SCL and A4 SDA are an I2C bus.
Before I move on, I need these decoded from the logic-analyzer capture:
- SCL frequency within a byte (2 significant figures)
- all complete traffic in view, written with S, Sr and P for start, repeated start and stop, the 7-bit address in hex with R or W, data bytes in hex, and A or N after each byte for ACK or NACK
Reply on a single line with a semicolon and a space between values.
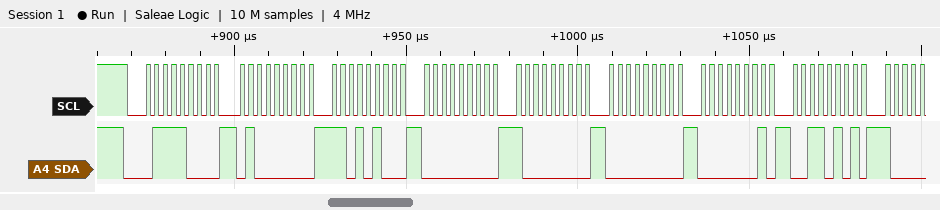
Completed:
400 kHz; S 3CW A 40 A D4 A 00 A 80 A 00 A 01 A 35 A
